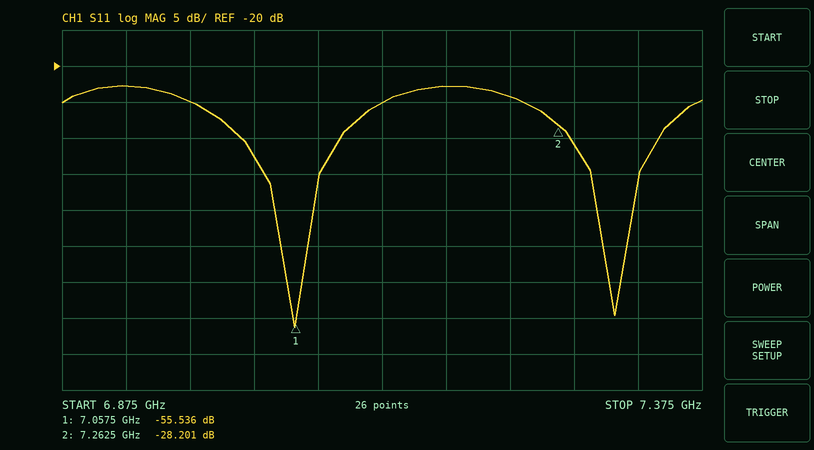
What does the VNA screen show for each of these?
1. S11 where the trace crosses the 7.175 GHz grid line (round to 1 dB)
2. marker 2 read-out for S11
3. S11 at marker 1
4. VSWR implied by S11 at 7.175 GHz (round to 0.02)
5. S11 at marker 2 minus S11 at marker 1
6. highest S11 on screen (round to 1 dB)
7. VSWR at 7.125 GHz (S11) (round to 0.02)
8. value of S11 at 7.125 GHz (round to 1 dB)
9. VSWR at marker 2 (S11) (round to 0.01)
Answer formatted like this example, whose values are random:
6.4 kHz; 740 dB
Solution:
-23 dB; -28.201 dB; -55.536 dB; 1.16; 27.335 dB; -23 dB; 1.12; -25 dB; 1.08
